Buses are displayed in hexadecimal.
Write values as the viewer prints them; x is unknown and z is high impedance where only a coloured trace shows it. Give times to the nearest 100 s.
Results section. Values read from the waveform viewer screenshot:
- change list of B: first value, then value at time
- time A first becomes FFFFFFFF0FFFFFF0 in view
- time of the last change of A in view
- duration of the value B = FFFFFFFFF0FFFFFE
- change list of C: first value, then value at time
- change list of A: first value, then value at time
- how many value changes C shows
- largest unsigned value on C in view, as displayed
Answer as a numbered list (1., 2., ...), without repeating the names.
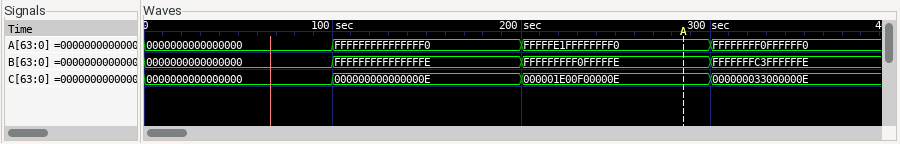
1. 0000000000000000, FFFFFFFFFFFFFFFE at 100 s, FFFFFFFFF0FFFFFE at 200 s, FFFFFFFC3FFFFFFE at 300 s
2. 300 s
3. 300 s
4. 100 s
5. 0000000000000000, 000000000000000E at 100 s, 000001E00F00000E at 200 s, 000000033000000E at 300 s
6. 0000000000000000, FFFFFFFFFFFFFFF0 at 100 s, FFFFFE1FFFFFFFF0 at 200 s, FFFFFFFF0FFFFFF0 at 300 s
7. 3
8. 000001E00F00000E
